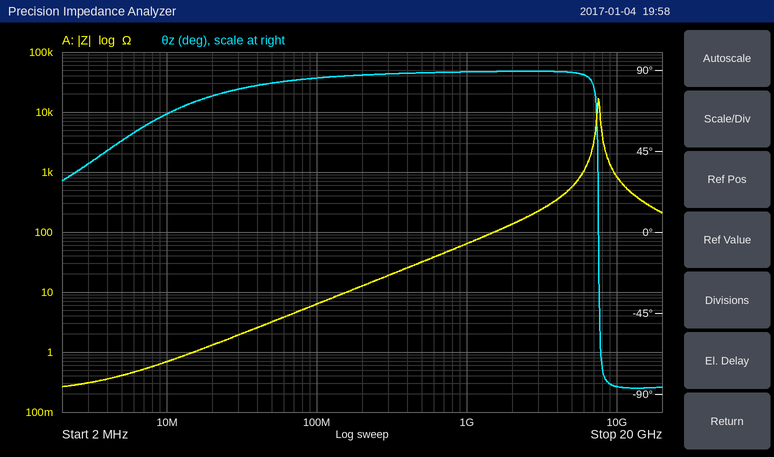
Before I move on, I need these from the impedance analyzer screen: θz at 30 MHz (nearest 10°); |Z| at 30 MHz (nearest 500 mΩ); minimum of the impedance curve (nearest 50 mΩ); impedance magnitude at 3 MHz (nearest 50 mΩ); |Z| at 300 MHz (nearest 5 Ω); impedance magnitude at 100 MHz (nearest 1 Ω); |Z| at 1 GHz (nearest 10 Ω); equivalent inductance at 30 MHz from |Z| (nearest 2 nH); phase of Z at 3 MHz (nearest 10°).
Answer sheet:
80°
2.0 Ω
250 mΩ
300 mΩ
20 Ω
6 Ω
60 Ω
10 nH
40°
